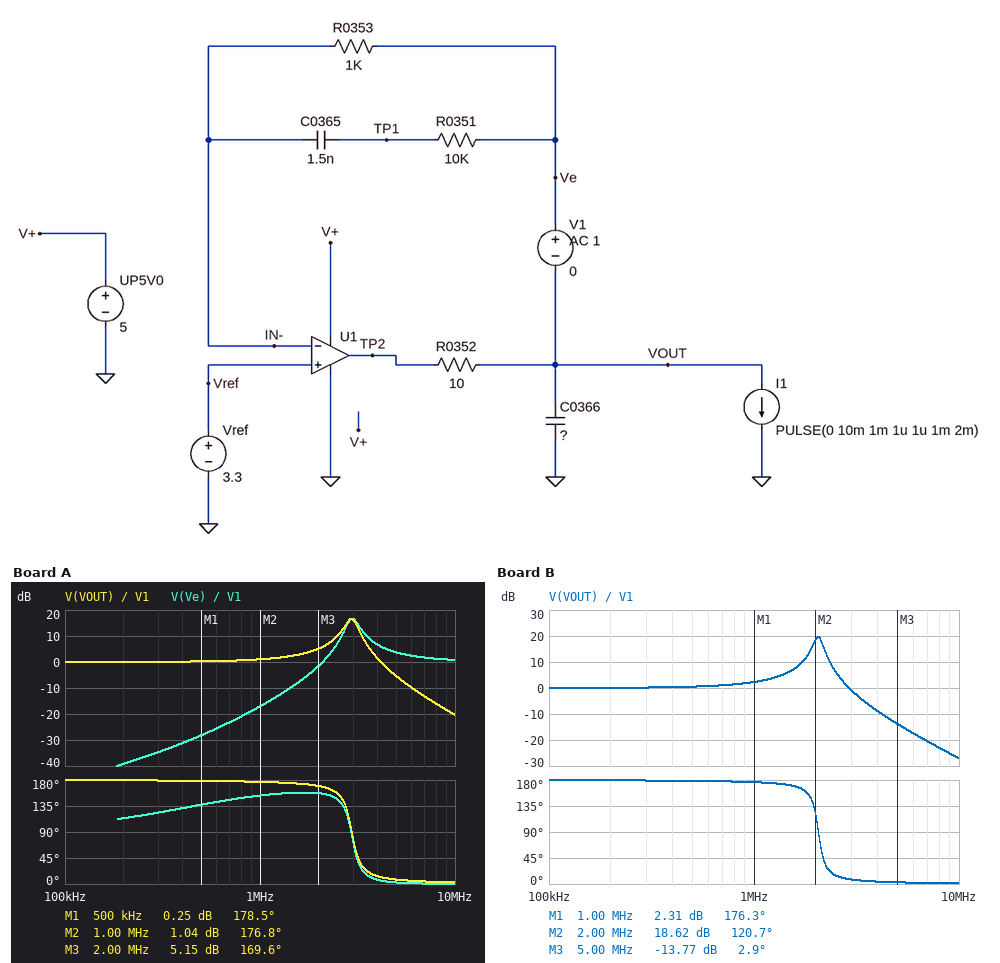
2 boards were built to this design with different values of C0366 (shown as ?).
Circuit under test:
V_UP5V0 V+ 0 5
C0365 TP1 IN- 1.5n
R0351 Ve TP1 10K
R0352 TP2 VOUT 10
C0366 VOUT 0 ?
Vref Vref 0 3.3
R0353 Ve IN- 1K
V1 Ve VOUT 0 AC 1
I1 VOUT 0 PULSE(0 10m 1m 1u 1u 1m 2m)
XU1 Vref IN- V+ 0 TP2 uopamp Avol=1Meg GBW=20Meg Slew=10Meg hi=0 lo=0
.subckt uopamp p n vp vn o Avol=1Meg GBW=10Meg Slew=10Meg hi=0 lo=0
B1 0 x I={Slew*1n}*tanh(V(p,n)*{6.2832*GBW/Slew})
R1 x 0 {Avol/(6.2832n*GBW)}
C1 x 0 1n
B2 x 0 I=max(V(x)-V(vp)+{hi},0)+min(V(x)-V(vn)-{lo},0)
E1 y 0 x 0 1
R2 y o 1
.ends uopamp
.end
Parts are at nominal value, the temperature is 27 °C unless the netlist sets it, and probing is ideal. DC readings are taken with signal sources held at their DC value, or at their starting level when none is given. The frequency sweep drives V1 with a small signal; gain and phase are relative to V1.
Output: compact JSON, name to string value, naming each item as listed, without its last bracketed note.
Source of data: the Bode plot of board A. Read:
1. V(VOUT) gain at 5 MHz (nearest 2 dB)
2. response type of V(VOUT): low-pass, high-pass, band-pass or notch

{"V(VOUT) gain at 5 MHz": "-6 dB", "response type of V(VOUT): low-pass, high-pass, band-pass or notch": "low-pass"}
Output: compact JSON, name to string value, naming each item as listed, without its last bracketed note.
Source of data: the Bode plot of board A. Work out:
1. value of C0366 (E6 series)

{"value of C0366": "33 nF"}
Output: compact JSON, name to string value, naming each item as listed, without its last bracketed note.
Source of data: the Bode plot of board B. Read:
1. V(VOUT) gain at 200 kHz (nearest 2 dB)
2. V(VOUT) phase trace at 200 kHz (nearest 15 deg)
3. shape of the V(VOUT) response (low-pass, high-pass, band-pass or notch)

{"V(VOUT) gain at 200 kHz": "0 dB", "V(VOUT) phase trace at 200 kHz": "180 deg", "shape of the V(VOUT) response": "low-pass"}
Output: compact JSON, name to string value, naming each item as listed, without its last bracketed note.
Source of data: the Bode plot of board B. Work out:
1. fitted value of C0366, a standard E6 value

{"fitted value of C0366, a standard E6 value": "68 nF"}
